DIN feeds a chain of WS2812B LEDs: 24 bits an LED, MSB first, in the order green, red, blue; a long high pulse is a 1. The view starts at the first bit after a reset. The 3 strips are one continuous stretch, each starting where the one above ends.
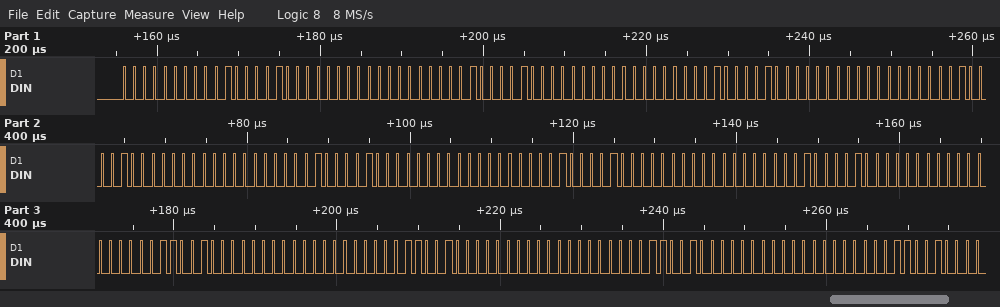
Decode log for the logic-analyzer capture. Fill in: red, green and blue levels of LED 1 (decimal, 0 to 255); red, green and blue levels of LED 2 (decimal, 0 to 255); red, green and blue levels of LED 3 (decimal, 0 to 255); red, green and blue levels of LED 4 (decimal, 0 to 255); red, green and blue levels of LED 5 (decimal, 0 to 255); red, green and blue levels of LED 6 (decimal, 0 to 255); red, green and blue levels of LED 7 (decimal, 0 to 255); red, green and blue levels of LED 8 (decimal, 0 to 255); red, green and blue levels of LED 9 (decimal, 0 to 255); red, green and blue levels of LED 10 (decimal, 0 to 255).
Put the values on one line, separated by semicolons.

33, 0, 0; 33, 0, 0; 33, 0, 0; 33, 0, 0; 33, 0, 0; 33, 0, 0; 33, 0, 0; 50, 0, 0; 50, 0, 0; 50, 0, 0
